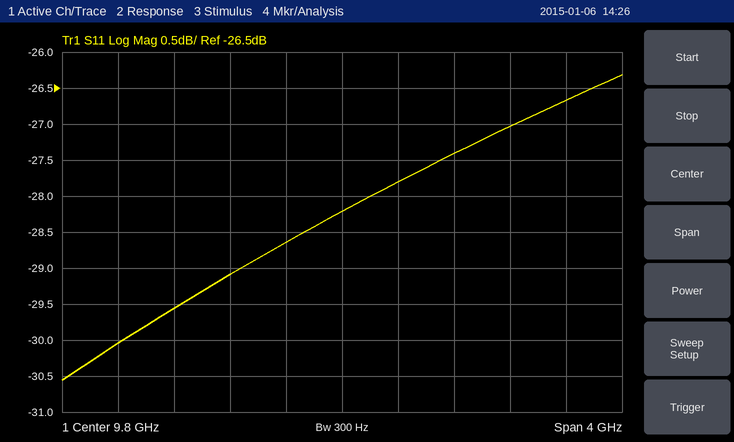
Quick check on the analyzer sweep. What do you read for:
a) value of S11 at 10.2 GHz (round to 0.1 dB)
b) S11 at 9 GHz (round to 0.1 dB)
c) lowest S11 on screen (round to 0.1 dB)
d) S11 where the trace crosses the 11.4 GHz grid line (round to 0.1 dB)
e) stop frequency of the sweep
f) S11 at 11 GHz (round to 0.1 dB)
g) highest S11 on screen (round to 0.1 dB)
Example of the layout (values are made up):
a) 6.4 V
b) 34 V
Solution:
a) -27.8 dB
b) -29.1 dB
c) -30.6 dB
d) -26.7 dB
e) 11.8 GHz
f) -27.0 dB
g) -26.3 dB
